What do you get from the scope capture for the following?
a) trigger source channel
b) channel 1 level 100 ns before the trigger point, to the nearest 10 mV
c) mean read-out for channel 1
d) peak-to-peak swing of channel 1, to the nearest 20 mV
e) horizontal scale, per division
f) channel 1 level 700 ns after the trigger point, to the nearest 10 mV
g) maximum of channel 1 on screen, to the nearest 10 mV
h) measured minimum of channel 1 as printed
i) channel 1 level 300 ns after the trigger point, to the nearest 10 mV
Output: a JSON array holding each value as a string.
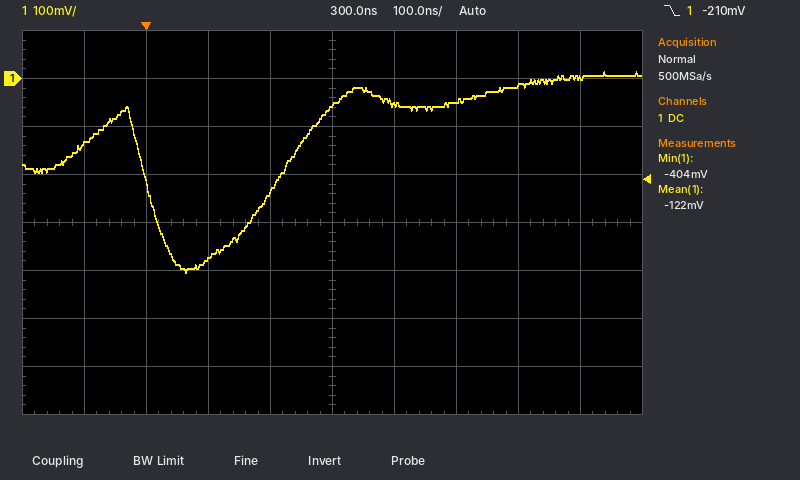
["channel 1", "-140 mV", "-122 mV", "420 mV", "100 ns", "0 mV", "10 mV", "-404 mV", "-60 mV"]
